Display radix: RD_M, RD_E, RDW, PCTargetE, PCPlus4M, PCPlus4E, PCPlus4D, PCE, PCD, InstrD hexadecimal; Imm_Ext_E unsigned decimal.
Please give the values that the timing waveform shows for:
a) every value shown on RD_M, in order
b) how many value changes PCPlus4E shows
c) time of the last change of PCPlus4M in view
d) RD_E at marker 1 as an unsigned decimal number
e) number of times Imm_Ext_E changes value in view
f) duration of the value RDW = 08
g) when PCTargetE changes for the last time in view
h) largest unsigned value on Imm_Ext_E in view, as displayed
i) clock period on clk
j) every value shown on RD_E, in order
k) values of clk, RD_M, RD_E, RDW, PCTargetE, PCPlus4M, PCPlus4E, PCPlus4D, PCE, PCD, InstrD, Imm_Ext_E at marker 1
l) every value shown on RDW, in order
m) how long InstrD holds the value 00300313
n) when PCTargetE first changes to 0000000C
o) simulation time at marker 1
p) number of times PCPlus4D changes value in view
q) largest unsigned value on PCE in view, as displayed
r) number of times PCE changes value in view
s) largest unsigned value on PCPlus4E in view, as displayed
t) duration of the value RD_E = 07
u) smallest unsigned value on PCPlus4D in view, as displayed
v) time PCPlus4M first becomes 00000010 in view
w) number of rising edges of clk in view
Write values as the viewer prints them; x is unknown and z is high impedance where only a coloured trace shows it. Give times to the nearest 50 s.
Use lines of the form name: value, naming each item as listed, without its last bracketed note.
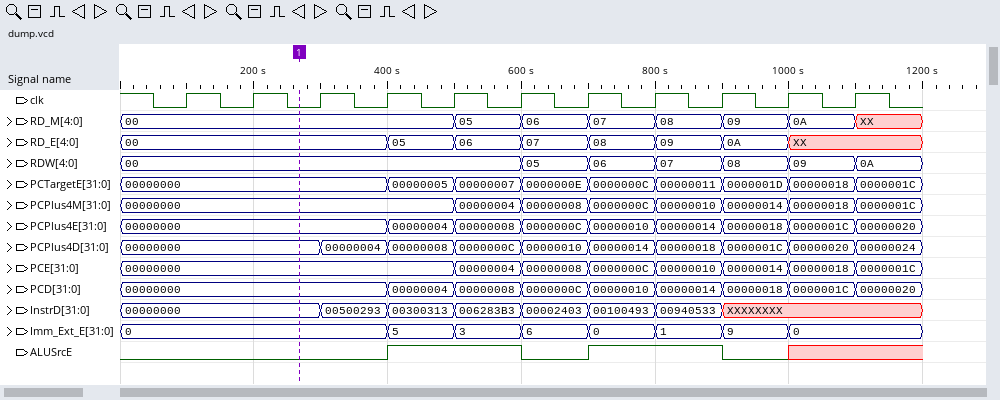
every value shown on RD_M, in order: 00, 05, 06, 07, 08, 09, 0A, XX
how many value changes PCPlus4E shows: 8
time of the last change of PCPlus4M in view: 1100 s
RD_E at marker 1 as an unsigned decimal number: 0
number of times Imm_Ext_E changes value in view: 7
duration of the value RDW = 08: 100 s
when PCTargetE changes for the last time in view: 1100 s
largest unsigned value on Imm_Ext_E in view, as displayed: 9
clock period on clk: 100 s
every value shown on RD_E, in order: 00, 05, 06, 07, 08, 09, 0A, XX
values of clk, RD_M, RD_E, RDW, PCTargetE, PCPlus4M, PCPlus4E, PCPlus4D, PCE, PCD, InstrD, Imm_Ext_E at marker 1: clk=0, RD_M=00, RD_E=00, RDW=00, PCTargetE=00000000, PCPlus4M=00000000, PCPlus4E=00000000, PCPlus4D=00000000, PCE=00000000, PCD=00000000, InstrD=00000000, Imm_Ext_E=0
every value shown on RDW, in order: 00, 05, 06, 07, 08, 09, 0A
how long InstrD holds the value 00300313: 100 s
when PCTargetE first changes to 0000000C: 700 s
simulation time at marker 1: 250 s
number of times PCPlus4D changes value in view: 9
largest unsigned value on PCE in view, as displayed: 0000001C
number of times PCE changes value in view: 7
largest unsigned value on PCPlus4E in view, as displayed: 00000020
duration of the value RD_E = 07: 100 s
smallest unsigned value on PCPlus4D in view, as displayed: 00000000
time PCPlus4M first becomes 00000010 in view: 800 s
number of rising edges of clk in view: 11
